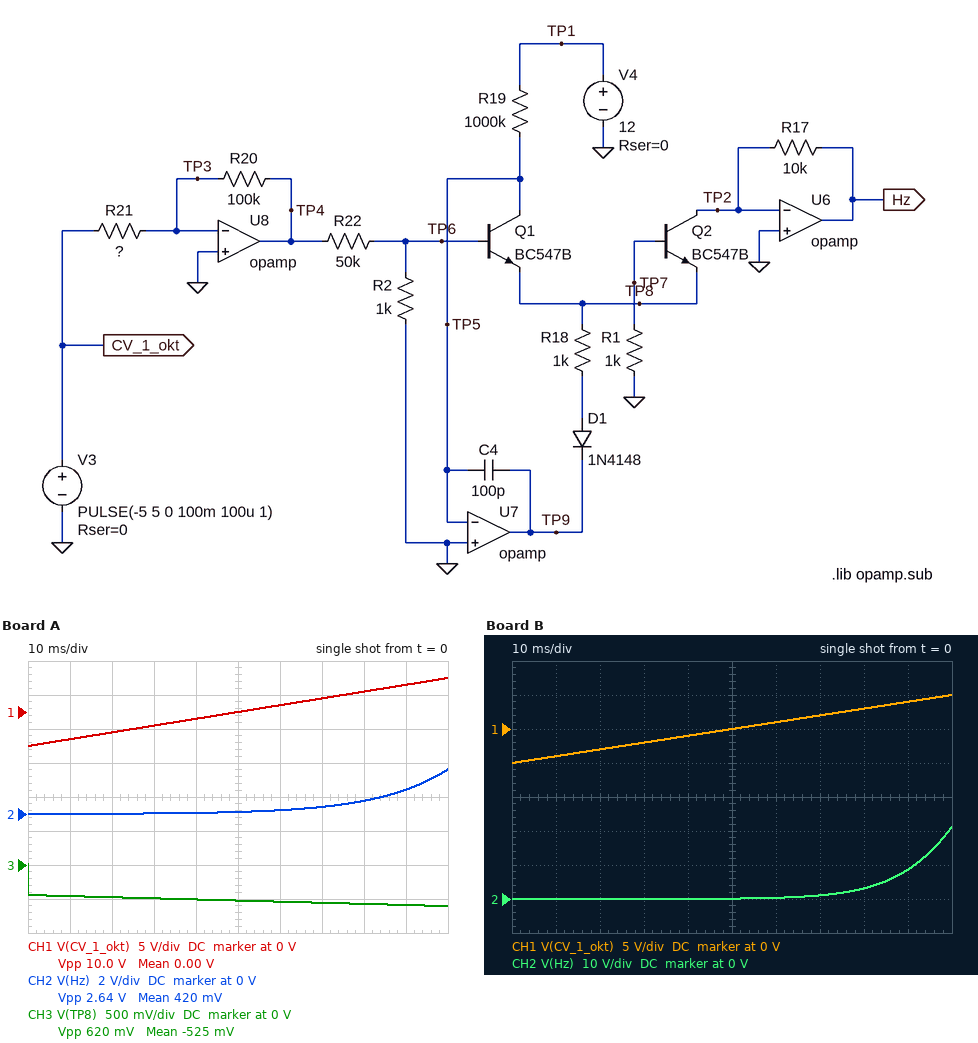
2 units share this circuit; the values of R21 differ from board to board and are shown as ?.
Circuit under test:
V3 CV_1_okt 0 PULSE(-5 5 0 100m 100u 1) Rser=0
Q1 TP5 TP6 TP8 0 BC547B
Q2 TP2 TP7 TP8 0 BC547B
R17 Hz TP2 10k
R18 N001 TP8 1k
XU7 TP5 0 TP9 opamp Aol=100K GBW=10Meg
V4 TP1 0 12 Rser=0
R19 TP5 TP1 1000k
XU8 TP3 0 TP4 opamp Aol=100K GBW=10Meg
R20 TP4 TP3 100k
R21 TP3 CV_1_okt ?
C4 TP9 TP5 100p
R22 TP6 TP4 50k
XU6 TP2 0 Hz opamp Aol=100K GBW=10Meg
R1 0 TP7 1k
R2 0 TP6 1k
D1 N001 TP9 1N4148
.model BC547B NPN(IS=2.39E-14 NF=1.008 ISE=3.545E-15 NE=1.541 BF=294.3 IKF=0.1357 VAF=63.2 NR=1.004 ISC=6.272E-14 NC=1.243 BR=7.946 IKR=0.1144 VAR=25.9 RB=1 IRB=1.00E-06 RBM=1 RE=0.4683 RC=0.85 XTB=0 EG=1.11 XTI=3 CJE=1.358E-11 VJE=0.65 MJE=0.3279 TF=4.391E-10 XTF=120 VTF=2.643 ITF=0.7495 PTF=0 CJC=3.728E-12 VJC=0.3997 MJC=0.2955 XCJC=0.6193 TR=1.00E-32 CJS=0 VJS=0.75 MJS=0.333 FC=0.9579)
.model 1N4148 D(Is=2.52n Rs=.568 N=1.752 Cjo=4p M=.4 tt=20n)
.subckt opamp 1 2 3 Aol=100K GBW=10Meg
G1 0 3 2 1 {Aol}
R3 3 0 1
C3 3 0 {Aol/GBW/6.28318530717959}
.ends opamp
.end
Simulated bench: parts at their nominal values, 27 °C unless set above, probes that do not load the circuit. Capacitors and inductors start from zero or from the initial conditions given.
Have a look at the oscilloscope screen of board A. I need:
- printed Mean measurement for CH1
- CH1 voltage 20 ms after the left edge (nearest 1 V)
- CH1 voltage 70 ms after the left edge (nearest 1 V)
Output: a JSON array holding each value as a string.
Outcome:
["0.00 V", "-3 V", "2 V"]
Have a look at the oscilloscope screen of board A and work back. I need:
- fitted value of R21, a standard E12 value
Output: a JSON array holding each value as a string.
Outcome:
["120 kΩ"]
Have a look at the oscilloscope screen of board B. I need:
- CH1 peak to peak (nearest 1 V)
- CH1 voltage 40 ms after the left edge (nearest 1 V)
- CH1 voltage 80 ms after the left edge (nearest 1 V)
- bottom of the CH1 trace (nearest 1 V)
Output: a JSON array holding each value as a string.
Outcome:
["10 V", "-1 V", "3 V", "-5 V"]
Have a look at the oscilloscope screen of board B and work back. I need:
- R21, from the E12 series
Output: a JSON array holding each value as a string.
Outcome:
["68 kΩ"]
